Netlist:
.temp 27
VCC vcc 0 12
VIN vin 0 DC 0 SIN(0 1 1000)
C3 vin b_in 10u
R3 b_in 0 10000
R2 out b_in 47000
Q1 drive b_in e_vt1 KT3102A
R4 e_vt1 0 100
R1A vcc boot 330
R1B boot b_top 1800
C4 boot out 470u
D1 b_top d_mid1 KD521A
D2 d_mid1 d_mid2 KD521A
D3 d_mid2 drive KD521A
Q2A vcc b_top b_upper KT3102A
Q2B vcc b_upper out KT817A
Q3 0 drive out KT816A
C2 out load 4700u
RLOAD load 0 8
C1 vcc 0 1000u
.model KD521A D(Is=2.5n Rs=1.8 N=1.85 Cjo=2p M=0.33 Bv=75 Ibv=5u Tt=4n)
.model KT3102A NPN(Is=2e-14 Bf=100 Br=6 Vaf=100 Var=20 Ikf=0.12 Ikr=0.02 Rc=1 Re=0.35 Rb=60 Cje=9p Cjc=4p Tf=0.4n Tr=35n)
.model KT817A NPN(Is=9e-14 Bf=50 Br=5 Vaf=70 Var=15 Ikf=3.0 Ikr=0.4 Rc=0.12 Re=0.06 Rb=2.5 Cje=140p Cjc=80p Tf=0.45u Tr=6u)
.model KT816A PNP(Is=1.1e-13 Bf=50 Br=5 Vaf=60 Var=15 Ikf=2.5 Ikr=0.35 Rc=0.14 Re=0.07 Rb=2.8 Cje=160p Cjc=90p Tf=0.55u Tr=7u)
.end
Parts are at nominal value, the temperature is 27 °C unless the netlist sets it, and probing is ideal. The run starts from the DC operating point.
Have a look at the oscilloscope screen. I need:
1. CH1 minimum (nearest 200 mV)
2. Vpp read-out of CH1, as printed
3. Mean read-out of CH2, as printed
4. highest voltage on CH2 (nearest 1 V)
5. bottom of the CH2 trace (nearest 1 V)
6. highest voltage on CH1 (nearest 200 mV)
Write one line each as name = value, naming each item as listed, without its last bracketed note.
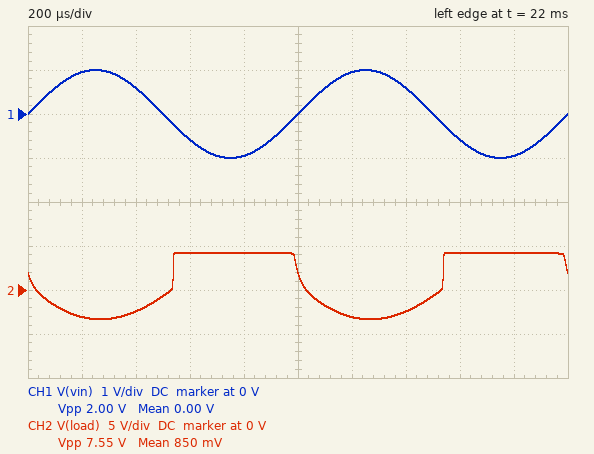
CH1 minimum = -1.0 V
Vpp read-out of CH1, as printed = 2.00 V
Mean read-out of CH2, as printed = 850 mV
highest voltage on CH2 = 4 V
bottom of the CH2 trace = -3 V
highest voltage on CH1 = 1.0 V
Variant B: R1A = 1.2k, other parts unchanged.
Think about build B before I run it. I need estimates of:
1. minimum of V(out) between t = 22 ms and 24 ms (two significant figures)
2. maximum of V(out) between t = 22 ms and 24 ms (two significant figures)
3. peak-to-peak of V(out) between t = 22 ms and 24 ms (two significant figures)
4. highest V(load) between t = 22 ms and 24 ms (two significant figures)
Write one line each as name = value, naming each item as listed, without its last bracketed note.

minimum of V(out) between t = 22 ms and 24 ms = 3.2 V
maximum of V(out) between t = 22 ms and 24 ms = 11 V
peak-to-peak of V(out) between t = 22 ms and 24 ms = 7.9 V
highest V(load) between t = 22 ms and 24 ms = 4.6 V
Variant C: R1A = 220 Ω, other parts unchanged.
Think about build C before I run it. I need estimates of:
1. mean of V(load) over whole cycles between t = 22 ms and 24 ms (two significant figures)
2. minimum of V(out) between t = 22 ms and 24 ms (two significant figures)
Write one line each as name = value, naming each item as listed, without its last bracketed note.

mean of V(load) over whole cycles between t = 22 ms and 24 ms = 800 mV
minimum of V(out) between t = 22 ms and 24 ms = 3.7 V
